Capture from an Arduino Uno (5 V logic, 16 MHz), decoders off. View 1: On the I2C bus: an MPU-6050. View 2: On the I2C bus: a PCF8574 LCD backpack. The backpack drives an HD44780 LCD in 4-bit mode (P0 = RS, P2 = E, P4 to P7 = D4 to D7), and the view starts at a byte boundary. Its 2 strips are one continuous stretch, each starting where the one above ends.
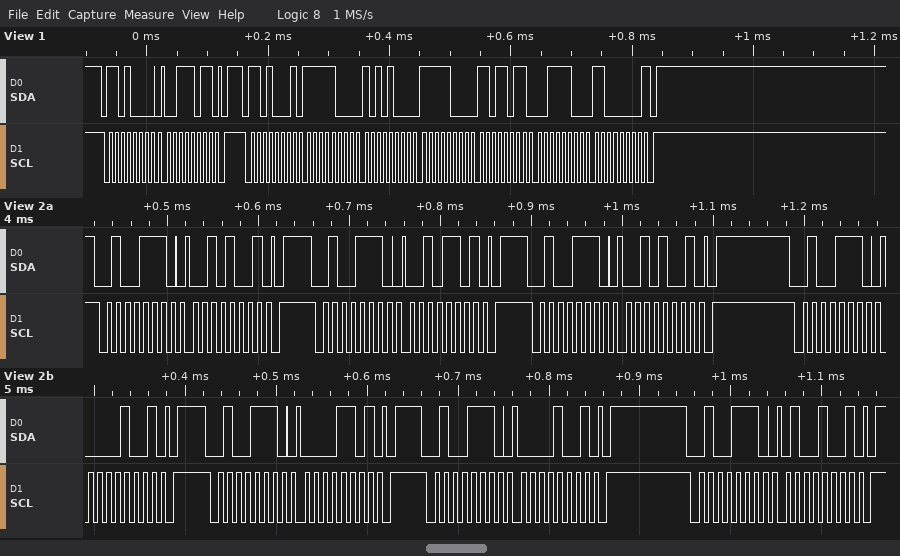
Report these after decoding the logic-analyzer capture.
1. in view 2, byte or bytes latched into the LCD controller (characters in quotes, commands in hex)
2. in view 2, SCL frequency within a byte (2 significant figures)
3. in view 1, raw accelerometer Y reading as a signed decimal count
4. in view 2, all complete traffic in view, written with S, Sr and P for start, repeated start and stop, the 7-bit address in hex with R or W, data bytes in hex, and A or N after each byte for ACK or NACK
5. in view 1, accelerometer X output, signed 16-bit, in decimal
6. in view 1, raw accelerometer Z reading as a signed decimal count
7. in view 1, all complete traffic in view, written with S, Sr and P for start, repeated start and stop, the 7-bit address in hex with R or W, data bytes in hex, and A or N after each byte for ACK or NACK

' '
100 kHz
-1829
S 27W A 29 A P S 27W A 2D A P S 27W A 29 A P S 27W A 09 A P S 27W A 0D A P S 27W A 09 A P S 27W A 49 A P
-1880
15552
S 68W A 3B A P S 68R A F8 A A8 A F8 A DB A 3C A C0 N P
